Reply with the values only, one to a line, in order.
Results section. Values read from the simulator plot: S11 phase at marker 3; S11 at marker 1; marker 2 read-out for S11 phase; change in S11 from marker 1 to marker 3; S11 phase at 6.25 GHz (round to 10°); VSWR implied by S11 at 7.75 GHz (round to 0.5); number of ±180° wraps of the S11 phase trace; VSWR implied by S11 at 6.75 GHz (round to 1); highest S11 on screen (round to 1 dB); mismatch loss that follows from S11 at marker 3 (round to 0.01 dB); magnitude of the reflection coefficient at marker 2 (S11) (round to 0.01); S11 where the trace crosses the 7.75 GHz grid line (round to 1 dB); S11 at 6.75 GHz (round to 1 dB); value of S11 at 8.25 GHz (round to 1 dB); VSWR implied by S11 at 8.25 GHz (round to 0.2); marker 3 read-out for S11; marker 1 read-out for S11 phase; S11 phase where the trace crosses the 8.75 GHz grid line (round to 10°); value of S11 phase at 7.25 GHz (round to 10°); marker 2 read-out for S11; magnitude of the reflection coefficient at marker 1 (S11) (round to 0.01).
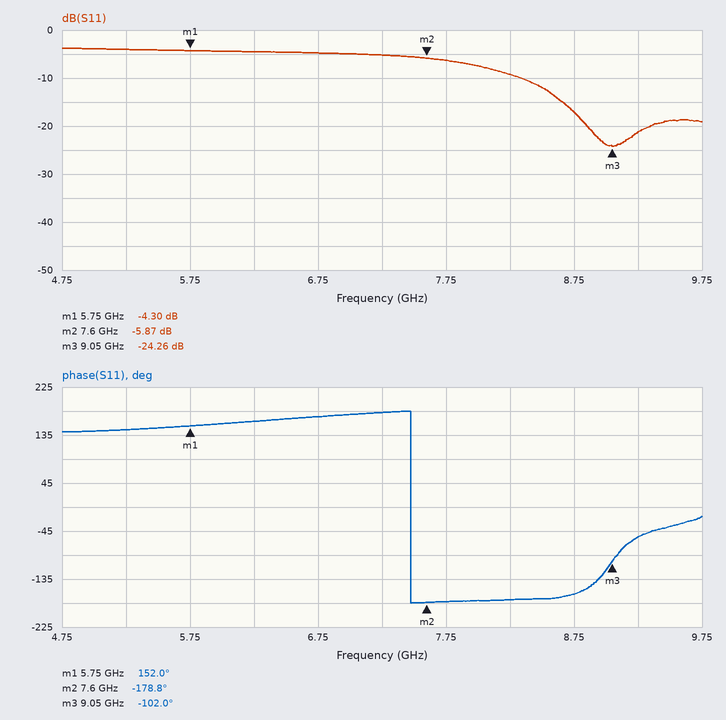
-102.0°
-4.30 dB
-178.8°
-19.96 dB
160°
3.0
1
4
-4 dB
0.02 dB
0.51
-6 dB
-5 dB
-9 dB
2.0
-24.26 dB
152.0°
-160°
180°
-5.87 dB
0.61
